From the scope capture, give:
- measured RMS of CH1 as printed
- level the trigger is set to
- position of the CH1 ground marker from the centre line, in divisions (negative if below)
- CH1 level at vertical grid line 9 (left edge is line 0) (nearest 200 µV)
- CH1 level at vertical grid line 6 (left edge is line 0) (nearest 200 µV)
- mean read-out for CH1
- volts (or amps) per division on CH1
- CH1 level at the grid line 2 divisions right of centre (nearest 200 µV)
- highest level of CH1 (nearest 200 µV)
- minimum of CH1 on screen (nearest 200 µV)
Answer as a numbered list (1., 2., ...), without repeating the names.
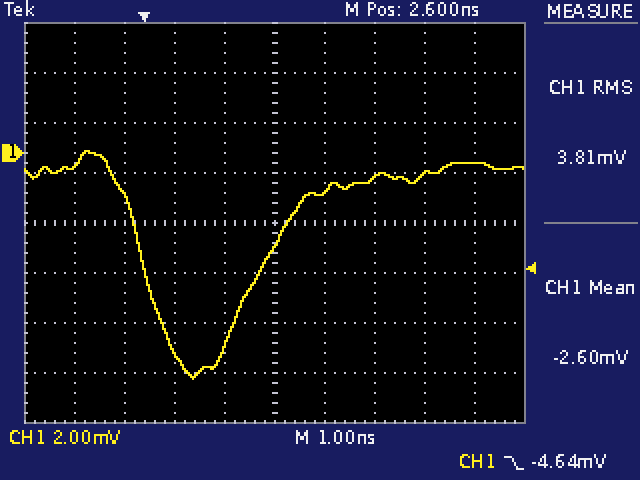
1. 3.81 mV
2. -4.64 mV
3. +1.4 div
4. -400 µV
5. -1.6 mV
6. -2.60 mV
7. 2 mV
8. -1.0 mV
9. 0.0 mV
10. -9.0 mV
